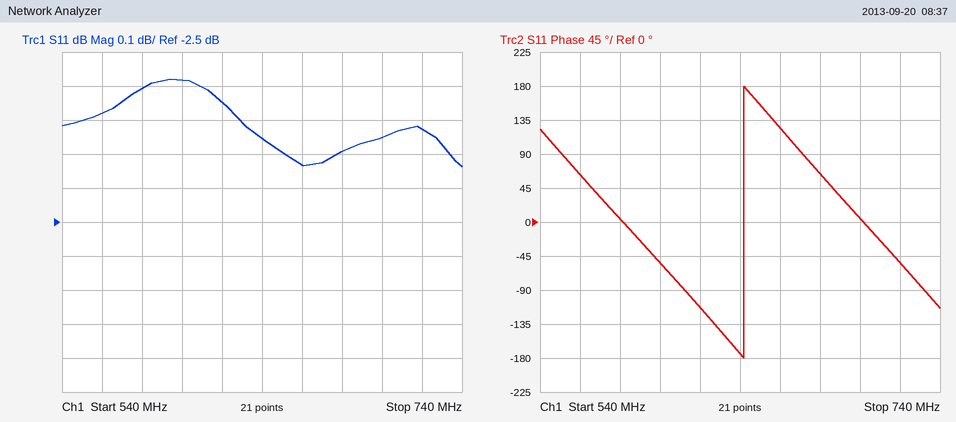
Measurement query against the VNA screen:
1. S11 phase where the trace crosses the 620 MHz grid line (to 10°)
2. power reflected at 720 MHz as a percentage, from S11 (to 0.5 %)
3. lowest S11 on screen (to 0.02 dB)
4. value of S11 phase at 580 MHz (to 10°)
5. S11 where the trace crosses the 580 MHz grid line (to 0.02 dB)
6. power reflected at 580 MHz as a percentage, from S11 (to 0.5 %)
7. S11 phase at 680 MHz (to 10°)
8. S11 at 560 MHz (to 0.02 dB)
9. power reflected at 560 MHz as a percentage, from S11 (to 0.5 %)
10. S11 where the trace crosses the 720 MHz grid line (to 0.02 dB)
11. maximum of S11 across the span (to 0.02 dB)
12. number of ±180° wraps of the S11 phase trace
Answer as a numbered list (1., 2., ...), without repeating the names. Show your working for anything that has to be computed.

1. -110°
2. 10^(-2.22/10) ≈ 60.0 %
3. -2.34 dB
4. 0°
5. -2.10 dB
6. 10^(-2.1/10) ≈ 61.7 %, so 61.5 % to the nearest 0.5 %
7. 60°
8. -2.18 dB
9. 10^(-2.18/10) ≈ 60.5 %
10. -2.22 dB
11. -2.08 dB
12. 1
